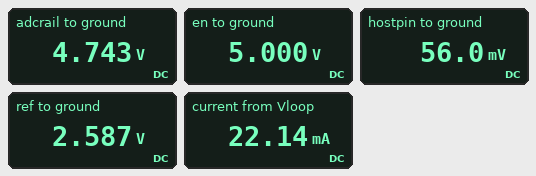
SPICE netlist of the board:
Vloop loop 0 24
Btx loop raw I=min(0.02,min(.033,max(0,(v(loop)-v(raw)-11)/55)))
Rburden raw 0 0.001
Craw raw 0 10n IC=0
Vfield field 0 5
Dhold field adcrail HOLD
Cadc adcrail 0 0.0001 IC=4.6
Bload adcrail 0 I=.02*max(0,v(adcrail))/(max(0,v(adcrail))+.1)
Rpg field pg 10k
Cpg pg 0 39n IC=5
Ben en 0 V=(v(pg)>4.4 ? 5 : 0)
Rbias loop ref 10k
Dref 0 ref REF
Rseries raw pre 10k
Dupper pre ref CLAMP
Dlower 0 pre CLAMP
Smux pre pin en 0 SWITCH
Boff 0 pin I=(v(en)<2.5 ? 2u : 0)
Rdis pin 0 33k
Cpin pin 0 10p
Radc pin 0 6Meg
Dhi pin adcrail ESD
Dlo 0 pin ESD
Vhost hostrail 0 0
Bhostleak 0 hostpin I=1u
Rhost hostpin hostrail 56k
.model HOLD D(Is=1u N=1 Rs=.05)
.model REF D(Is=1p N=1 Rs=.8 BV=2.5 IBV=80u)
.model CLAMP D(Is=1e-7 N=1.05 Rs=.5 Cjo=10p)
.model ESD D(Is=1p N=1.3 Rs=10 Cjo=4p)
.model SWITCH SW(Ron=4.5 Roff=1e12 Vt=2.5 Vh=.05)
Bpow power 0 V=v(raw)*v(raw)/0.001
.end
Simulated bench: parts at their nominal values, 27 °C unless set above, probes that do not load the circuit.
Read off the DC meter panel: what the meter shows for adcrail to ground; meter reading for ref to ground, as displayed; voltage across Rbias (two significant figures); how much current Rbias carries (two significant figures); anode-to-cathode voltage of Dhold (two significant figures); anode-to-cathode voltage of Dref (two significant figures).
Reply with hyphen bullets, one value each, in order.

- 4.743 V
- 2.587 V
- 21 V
- 2.1 mA
- 260 mV
- -2.6 V
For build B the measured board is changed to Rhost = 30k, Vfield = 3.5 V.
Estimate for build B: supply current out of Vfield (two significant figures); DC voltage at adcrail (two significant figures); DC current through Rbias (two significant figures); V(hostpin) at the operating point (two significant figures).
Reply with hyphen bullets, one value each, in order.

- 19 mA
- 3.2 V
- 2.1 mA
- 30 mV
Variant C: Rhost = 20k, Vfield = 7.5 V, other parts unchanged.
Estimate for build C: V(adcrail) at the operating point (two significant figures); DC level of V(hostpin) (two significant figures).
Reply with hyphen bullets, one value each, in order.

- 7.2 V
- 20 mV
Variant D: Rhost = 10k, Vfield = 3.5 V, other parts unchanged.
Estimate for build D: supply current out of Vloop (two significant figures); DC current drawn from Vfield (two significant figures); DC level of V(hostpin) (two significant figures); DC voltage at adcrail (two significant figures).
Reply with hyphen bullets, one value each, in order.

- 22 mA
- 19 mA
- 10 mV
- 3.2 V
